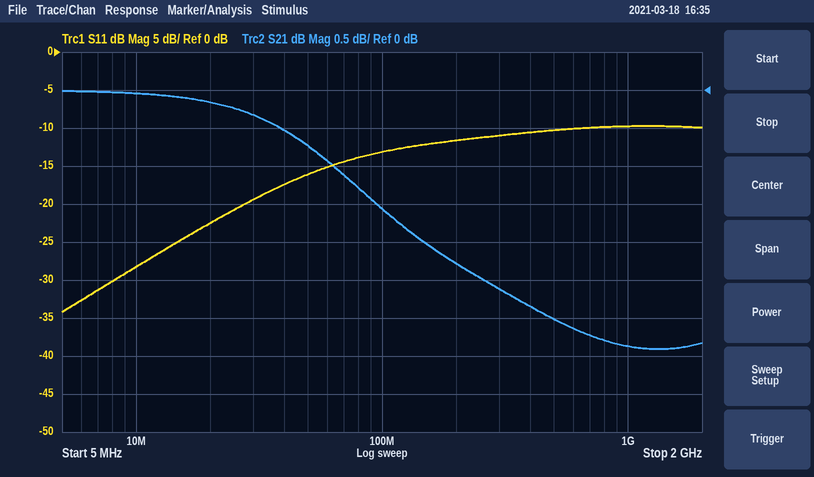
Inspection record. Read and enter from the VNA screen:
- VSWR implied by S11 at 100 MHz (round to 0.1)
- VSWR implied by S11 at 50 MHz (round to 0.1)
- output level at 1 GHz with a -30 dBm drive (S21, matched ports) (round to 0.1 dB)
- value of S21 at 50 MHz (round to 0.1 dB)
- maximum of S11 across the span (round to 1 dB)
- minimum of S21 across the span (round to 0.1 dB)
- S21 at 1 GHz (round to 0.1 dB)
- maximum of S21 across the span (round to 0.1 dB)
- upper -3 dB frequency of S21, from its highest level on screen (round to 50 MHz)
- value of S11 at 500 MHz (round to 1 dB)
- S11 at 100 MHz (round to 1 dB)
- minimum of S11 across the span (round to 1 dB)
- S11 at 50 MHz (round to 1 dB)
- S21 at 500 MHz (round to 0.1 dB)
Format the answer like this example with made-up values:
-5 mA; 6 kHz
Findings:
1.6; 1.4; -33.4 dBm; -0.7 dB; -10 dB; -3.4 dB; -3.4 dB; 0.0 dB; 500 MHz; -10 dB; -13 dB; -34 dB; -16 dB; -3.0 dB
